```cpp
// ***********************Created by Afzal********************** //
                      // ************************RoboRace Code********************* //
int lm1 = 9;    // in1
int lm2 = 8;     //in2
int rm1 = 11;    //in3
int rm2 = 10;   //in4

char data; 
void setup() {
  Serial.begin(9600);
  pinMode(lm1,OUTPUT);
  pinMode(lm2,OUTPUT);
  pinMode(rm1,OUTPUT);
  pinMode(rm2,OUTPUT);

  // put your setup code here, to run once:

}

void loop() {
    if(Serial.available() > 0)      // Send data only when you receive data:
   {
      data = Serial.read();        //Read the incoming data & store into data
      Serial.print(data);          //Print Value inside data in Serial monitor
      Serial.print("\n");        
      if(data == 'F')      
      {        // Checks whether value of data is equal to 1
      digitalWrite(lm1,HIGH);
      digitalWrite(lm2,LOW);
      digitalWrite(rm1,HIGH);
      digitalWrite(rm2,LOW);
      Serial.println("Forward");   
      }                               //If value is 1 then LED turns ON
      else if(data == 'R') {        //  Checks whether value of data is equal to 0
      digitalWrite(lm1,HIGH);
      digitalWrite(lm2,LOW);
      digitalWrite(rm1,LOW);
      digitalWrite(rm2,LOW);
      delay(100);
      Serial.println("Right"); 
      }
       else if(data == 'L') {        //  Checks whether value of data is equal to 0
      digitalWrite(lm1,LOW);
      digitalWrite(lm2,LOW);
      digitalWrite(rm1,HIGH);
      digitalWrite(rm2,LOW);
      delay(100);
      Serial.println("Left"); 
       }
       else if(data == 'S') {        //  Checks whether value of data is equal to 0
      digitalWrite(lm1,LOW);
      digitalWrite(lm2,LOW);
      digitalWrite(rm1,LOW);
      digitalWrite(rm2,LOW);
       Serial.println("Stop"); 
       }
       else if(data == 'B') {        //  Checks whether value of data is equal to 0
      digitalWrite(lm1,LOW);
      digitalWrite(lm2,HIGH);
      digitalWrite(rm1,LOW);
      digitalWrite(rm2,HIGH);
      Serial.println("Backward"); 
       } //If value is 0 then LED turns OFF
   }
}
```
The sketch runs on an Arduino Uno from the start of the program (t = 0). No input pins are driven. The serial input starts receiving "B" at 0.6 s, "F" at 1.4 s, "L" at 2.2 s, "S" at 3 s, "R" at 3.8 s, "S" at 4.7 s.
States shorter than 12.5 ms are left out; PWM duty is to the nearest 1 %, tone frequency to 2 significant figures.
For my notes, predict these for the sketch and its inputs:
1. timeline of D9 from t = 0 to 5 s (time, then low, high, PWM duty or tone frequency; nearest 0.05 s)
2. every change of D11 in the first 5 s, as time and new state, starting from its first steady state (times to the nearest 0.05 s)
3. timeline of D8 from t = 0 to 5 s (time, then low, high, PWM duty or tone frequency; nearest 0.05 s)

0 s low; 1.4 s high; 2.2 s low; 3.8 s high; 4.7 s low
0 s low; 1.4 s high; 3 s low
0 s low; 0.6 s high; 1.4 s low
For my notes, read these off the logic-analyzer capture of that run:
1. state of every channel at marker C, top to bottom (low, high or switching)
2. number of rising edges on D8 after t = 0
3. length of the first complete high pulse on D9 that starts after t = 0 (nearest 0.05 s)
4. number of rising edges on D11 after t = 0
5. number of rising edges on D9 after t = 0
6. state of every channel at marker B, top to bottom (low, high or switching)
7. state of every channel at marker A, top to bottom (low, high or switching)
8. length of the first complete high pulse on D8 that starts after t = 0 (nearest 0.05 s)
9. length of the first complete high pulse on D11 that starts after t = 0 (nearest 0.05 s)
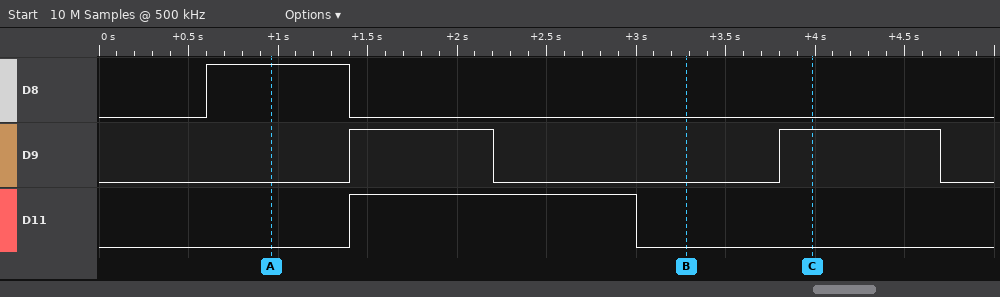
D8 low, D9 high, D11 low
1
0.80 s
1
2
D8 low, D9 low, D11 low
D8 high, D9 low, D11 low
0.80 s
1.60 s
